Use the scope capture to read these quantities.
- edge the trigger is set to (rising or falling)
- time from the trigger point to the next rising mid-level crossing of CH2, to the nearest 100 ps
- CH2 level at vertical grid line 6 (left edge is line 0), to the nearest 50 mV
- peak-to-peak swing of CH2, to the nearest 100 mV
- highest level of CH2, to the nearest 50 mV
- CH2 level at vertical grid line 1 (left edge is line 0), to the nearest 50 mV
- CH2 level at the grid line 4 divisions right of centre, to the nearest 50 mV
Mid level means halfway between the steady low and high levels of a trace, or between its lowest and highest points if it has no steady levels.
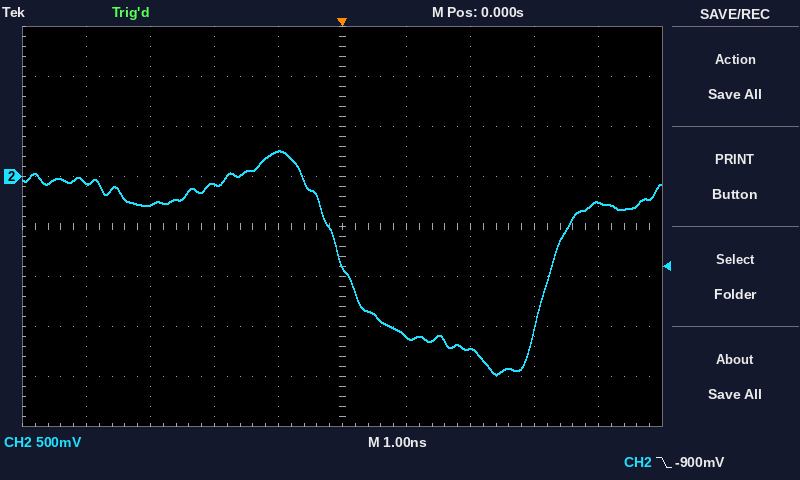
falling
3.3 ns
-1.60 V
2.20 V
250 mV
-50 mV
-250 mV
